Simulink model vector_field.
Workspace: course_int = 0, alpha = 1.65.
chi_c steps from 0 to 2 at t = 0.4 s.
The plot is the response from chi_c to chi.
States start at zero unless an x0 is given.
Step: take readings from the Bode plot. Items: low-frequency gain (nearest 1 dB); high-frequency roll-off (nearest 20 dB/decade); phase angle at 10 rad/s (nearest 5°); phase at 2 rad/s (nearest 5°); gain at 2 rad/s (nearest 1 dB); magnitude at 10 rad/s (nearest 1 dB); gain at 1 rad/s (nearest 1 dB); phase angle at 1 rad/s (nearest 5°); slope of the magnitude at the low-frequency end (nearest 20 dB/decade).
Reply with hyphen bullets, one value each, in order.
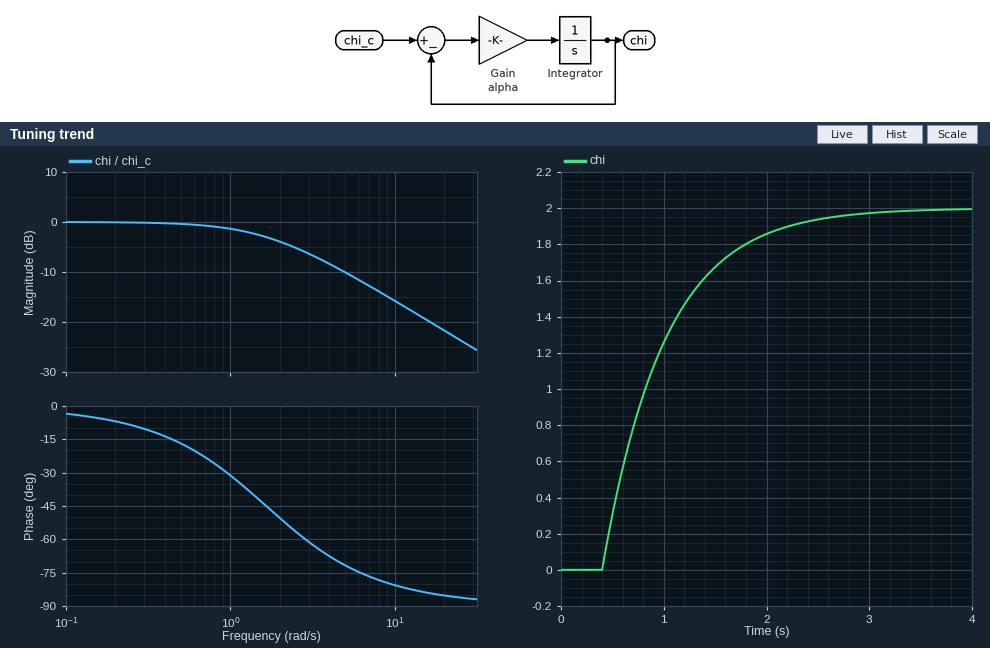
- 0 dB
- -20 dB/decade
- -80°
- -50°
- -4 dB
- -16 dB
- -1 dB
- -30°
- 0 dB/decade
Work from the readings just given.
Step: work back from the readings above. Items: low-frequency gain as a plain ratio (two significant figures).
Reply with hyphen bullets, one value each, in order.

- 1.0
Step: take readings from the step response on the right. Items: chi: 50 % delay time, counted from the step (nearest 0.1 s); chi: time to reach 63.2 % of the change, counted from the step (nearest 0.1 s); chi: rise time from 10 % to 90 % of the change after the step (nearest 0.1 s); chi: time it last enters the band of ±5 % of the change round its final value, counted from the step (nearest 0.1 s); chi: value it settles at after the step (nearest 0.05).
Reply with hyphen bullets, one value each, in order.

- 0.4 s
- 0.6 s
- 1.3 s
- 1.8 s
- 2.00
